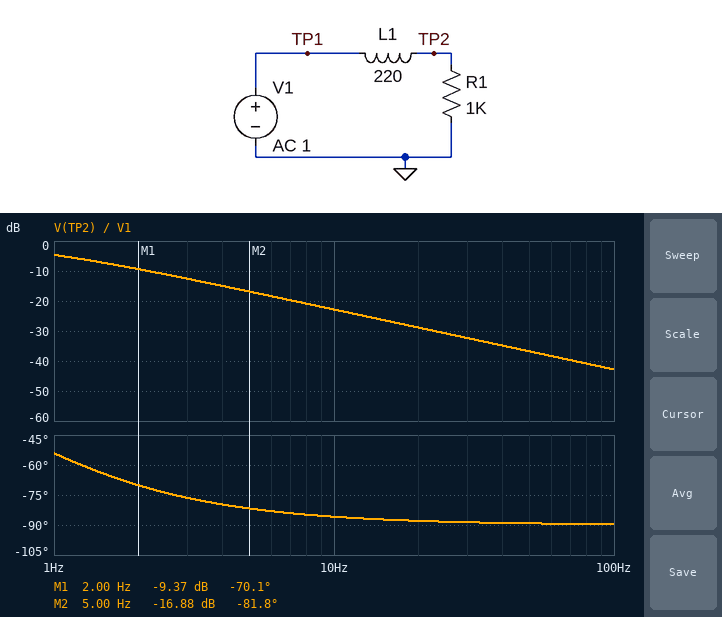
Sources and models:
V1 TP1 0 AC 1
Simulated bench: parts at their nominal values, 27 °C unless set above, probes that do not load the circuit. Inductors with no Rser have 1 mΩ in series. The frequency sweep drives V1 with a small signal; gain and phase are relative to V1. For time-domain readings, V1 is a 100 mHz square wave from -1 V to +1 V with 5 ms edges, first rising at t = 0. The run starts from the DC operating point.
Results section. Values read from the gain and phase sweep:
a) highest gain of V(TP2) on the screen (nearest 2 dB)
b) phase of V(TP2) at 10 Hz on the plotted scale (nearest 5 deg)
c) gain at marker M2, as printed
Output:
-4 dB
-85 deg
-16.88 dB
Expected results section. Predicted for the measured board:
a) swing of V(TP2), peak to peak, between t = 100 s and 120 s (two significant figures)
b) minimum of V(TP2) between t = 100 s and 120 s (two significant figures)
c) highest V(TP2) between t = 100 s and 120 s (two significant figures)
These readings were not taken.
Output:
2.0 V
-1.0 V
1.0 V
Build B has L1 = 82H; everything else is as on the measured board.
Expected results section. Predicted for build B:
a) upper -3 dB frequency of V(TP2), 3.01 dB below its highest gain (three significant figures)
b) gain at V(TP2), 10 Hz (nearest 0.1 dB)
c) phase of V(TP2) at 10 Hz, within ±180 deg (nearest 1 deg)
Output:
1.94 Hz
-14.4 dB
-79 deg
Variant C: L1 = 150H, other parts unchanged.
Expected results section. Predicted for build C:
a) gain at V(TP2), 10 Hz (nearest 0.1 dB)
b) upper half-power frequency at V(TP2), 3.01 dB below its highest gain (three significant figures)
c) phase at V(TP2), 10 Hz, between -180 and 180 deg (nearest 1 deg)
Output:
-19.5 dB
1.06 Hz
-84 deg
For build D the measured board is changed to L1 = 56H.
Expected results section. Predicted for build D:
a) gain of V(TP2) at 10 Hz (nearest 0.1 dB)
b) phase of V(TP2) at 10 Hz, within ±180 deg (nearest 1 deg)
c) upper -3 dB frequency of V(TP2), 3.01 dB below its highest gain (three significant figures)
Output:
-11.3 dB
-74 deg
2.84 Hz
